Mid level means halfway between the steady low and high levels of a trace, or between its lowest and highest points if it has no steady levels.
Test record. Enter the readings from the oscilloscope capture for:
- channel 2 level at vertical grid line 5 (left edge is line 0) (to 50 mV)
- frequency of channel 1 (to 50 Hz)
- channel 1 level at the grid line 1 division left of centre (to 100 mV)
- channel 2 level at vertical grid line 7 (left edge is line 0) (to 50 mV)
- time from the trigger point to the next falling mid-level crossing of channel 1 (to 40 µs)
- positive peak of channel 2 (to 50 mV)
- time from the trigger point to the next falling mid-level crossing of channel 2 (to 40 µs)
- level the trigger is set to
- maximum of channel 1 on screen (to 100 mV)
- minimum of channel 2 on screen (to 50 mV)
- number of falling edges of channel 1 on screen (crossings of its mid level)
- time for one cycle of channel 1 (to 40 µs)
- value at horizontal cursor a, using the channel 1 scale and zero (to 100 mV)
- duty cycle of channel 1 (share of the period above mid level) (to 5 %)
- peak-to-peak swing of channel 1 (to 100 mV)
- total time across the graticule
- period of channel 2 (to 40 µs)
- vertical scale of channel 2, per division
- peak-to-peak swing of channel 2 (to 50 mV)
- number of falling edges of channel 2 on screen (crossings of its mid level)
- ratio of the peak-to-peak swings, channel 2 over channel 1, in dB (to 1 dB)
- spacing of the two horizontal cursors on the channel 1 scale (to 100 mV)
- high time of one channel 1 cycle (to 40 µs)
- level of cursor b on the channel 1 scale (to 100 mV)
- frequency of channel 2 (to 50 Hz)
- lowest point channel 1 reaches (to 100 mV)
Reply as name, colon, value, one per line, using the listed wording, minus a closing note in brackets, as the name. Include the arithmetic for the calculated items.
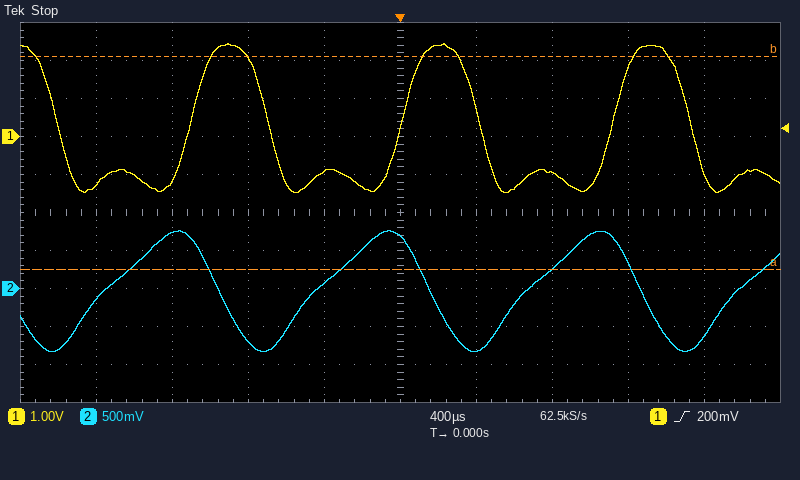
channel 2 level at vertical grid line 5 (left edge is line 0): 700 mV
frequency of channel 1: 1 / 1.12 ms ≈ 893 Hz, so 900 Hz to the nearest 50 Hz
channel 1 level at the grid line 1 division left of centre: -900 mV
channel 2 level at vertical grid line 7 (left edge is line 0): 250 mV
time from the trigger point to the next falling mid-level crossing of channel 1: 400 µs
positive peak of channel 2: 750 mV
time from the trigger point to the next falling mid-level crossing of channel 2: 160 µs
level the trigger is set to: 200 mV
maximum of channel 1 on screen: 2.4 V
minimum of channel 2 on screen: -850 mV
number of falling edges of channel 1 on screen: 4
time for one cycle of channel 1: 1.12 ms
value at horizontal cursor a, using the channel 1 scale and zero: -3.5 V
duty cycle of channel 1 (share of the period above mid level): 400 µs / 1.12 ms ≈ 35.7 %, so 35 % to the nearest 5 %
peak-to-peak swing of channel 1: 2.4 V − (-1.5 V) = 3.9 V
total time across the graticule: 4 ms
period of channel 2: 1.12 ms
vertical scale of channel 2, per division: 500 mV
peak-to-peak swing of channel 2: 750 mV − (-850 mV) = 1.60 V
number of falling edges of channel 2 on screen: 3
ratio of the peak-to-peak swings, channel 2 over channel 1, in dB: 20 log10(1.60 V / 3.9 V) ≈ -8 dB
spacing of the two horizontal cursors on the channel 1 scale: 5.6 V
high time of one channel 1 cycle: 400 µs
level of cursor b on the channel 1 scale: 2.1 V
frequency of channel 2: 1 / 1.12 ms ≈ 893 Hz, so 900 Hz to the nearest 50 Hz
lowest point channel 1 reaches: -1.5 V
